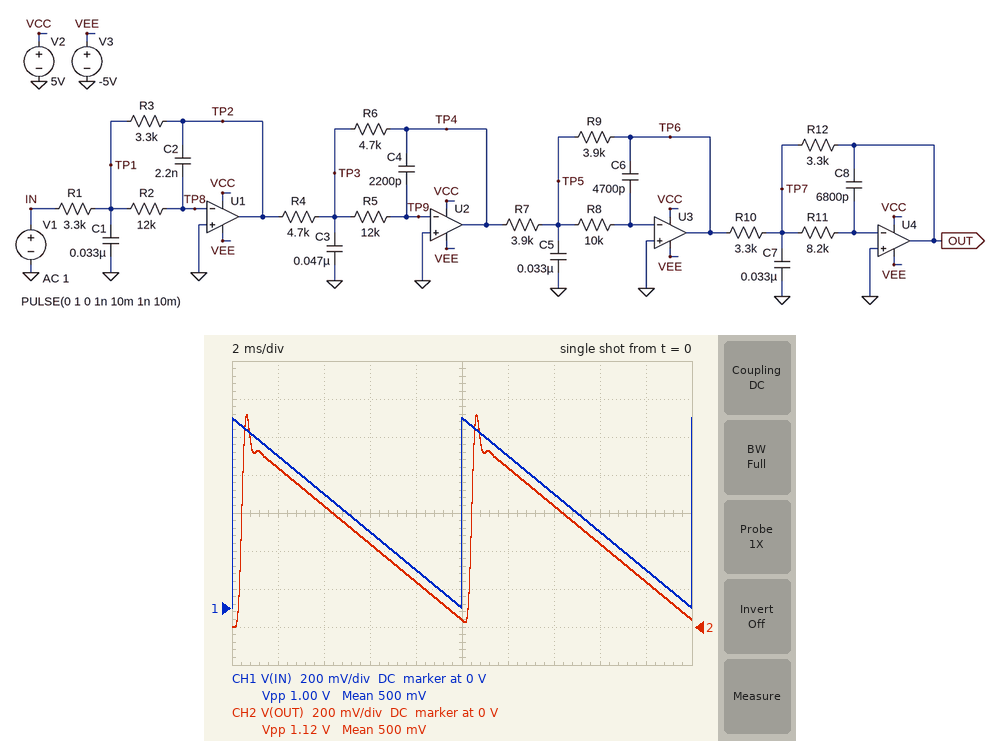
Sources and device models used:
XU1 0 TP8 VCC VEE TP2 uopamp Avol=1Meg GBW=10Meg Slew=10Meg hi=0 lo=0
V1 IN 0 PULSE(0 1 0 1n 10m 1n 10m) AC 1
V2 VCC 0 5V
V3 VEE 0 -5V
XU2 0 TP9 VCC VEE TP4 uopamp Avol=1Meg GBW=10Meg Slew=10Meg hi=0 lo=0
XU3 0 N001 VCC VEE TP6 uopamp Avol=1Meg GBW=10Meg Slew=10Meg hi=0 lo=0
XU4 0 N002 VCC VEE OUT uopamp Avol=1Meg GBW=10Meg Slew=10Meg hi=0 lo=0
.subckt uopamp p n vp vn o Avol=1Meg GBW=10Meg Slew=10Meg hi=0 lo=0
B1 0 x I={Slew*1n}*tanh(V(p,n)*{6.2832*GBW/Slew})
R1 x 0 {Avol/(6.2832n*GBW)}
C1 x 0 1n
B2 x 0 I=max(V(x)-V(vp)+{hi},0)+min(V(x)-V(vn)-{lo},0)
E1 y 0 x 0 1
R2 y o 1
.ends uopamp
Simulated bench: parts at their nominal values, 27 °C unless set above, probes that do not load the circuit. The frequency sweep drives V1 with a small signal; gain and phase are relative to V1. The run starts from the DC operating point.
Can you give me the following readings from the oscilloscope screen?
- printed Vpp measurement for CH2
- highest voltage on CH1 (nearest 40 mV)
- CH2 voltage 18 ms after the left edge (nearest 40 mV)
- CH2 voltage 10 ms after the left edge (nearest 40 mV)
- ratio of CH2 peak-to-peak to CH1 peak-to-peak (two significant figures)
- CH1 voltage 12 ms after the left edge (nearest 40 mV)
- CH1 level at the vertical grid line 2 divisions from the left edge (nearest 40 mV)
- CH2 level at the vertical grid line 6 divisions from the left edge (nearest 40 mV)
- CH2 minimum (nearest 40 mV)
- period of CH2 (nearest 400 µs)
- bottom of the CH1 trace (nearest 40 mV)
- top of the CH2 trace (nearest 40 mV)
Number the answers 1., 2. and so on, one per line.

1. 1.12 V
2. 1.00 V
3. 240 mV
4. 40 mV
5. 1.1
6. 800 mV
7. 600 mV
8. 840 mV
9. 0 V
10. 10.0 ms
11. 0 V
12. 1.12 V
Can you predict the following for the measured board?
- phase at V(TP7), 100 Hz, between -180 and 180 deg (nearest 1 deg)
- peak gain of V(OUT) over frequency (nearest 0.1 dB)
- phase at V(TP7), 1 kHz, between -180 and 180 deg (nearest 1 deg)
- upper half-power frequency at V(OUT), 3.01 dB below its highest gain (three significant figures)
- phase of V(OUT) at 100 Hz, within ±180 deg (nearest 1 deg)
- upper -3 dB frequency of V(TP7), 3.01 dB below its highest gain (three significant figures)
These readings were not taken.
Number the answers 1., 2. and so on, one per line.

1. -103 deg
2. 0.2 dB
3. 129 deg
4. 1.79 kHz
5. -13 deg
6. 2.16 kHz
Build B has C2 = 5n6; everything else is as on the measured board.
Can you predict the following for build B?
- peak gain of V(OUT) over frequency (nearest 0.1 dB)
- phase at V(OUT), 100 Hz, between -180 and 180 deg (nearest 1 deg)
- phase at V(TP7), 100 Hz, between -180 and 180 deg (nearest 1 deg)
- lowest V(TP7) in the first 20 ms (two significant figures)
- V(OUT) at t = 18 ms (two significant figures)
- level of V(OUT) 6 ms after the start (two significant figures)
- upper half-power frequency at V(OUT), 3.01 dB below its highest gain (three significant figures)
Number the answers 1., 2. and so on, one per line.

1. 0 dB
2. -17 deg
3. -107 deg
4. -180 mV
5. 250 mV
6. 450 mV
7. 1.25 kHz
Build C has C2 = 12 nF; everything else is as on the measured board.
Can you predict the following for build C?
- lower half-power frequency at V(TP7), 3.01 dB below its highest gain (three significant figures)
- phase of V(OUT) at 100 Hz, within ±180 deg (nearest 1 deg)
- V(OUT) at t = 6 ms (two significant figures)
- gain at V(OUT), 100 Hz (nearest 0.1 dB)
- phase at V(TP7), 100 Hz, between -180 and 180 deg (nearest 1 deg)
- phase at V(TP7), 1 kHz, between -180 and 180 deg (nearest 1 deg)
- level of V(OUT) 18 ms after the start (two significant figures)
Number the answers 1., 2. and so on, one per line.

1. 405 Hz
2. -23 deg
3. 460 mV
4. -0.1 dB
5. -113 deg
6. 72 deg
7. 260 mV
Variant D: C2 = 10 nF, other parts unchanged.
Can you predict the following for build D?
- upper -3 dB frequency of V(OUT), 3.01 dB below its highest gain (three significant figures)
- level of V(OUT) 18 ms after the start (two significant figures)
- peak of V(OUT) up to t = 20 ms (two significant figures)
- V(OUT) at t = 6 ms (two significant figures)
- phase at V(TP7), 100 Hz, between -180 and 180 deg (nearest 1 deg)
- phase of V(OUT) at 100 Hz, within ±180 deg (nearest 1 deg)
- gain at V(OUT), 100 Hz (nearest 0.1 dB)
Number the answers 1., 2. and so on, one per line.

1. 702 Hz
2. 260 mV
3. 920 mV
4. 460 mV
5. -111 deg
6. -21 deg
7. -0.1 dB
